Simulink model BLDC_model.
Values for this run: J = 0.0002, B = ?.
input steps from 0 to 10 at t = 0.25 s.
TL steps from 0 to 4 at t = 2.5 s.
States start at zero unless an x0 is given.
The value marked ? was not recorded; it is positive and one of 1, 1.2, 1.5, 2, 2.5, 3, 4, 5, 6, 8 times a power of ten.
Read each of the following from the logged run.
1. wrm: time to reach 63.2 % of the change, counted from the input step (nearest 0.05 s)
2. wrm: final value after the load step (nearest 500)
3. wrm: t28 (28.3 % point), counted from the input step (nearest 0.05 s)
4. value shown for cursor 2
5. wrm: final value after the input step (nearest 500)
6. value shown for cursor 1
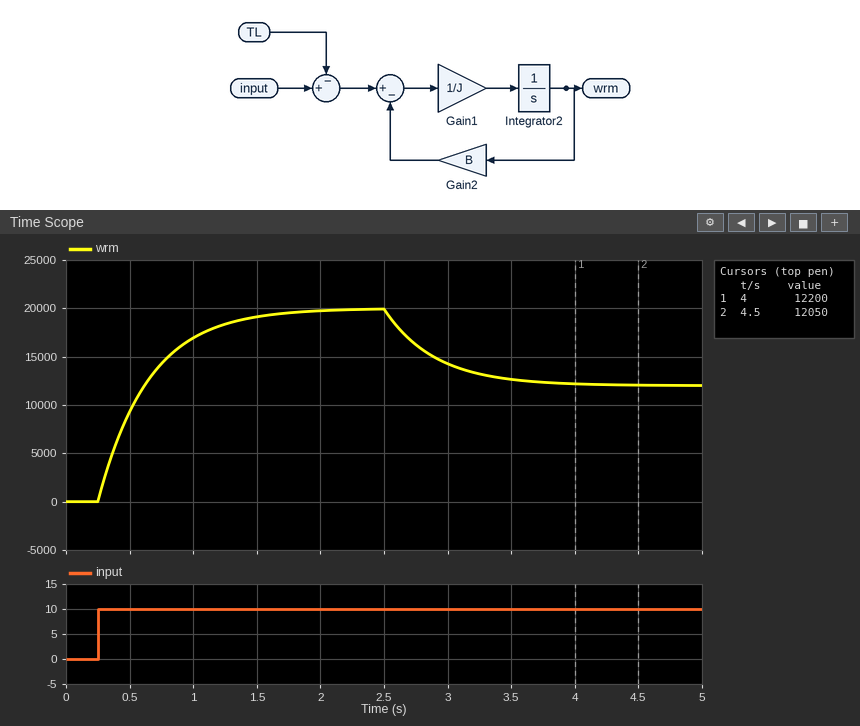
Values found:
0.40 s
12000
0.15 s
12050
20000
12200
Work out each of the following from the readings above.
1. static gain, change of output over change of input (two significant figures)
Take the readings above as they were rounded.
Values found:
2000
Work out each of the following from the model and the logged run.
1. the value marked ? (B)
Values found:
0.0005
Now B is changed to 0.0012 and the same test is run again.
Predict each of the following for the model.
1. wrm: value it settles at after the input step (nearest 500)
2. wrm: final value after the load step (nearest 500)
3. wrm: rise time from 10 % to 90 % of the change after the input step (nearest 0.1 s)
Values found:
8500
5000
0.4 s
